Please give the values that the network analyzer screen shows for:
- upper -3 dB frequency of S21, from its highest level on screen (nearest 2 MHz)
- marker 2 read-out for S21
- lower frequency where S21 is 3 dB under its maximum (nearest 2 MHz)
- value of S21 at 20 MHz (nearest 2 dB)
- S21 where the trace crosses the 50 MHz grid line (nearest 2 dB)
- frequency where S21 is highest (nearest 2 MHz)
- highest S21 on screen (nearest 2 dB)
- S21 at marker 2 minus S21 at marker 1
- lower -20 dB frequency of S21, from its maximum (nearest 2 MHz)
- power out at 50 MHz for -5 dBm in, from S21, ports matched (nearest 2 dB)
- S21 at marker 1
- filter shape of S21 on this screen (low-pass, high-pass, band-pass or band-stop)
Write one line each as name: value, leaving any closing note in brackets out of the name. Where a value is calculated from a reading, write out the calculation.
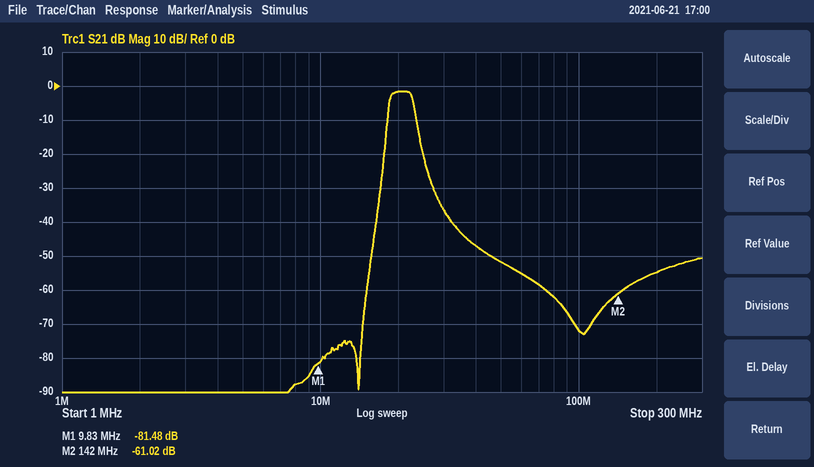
upper -3 dB frequency of S21, from its highest level on screen: 22 MHz
marker 2 read-out for S21: -61.02 dB
lower frequency where S21 is 3 dB under its maximum: 18 MHz
value of S21 at 20 MHz: -2 dB
S21 where the trace crosses the 50 MHz grid line: -52 dB
frequency where S21 is highest: 20 MHz
highest S21 on screen: -2 dB
S21 at marker 2 minus S21 at marker 1: -61.02 − (-81.48) = 20.46 dB
lower -20 dB frequency of S21, from its maximum: 18 MHz
power out at 50 MHz for -5 dBm in, from S21, ports matched: -5 dBm + (-52 dB) = -56 dBm
S21 at marker 1: -81.48 dB
filter shape of S21 on this screen: band-pass
